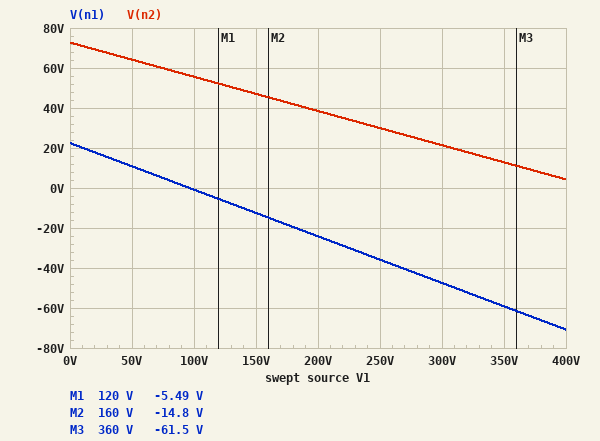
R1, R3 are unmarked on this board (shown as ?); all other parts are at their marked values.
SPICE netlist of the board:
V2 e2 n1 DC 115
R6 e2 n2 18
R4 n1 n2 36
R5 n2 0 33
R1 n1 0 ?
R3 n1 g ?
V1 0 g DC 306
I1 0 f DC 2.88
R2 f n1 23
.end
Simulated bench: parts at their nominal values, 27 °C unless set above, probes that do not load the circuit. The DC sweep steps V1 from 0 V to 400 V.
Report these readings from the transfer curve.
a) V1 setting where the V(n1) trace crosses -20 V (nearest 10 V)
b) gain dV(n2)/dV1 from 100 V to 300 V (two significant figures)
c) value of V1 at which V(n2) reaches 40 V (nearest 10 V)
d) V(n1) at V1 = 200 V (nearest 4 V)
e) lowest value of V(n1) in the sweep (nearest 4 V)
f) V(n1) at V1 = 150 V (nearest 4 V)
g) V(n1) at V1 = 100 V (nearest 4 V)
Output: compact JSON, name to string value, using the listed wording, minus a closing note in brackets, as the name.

{"V1 setting where the V(n1) trace crosses -20 V": "180 V", "gain dV(n2)/dV1 from 100 V to 300 V": "-0.17 V/V", "value of V1 at which V(n2) reaches 40 V": "190 V", "V(n1) at V1 = 200 V": "-24 V", "lowest value of V(n1) in the sweep": "-72 V", "V(n1) at V1 = 150 V": "-12 V", "V(n1) at V1 = 100 V": "0 V"}
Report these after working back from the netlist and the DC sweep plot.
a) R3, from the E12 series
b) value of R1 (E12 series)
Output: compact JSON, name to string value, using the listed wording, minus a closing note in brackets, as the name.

{"R3, from the E12 series": "82 Ω", "value of R1": "56 Ω"}
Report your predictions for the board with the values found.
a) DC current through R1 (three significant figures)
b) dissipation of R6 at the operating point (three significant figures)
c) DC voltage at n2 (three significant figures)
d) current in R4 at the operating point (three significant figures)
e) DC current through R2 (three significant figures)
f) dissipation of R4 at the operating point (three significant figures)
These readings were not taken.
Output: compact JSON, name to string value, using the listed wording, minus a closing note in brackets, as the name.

{"DC current through R1": "873 mA", "dissipation of R6 at the operating point": "116 W", "DC voltage at n2": "20.4 V", "current in R4 at the operating point": "1.92 A", "DC current through R2": "2.88 A", "dissipation of R4 at the operating point": "133 W"}
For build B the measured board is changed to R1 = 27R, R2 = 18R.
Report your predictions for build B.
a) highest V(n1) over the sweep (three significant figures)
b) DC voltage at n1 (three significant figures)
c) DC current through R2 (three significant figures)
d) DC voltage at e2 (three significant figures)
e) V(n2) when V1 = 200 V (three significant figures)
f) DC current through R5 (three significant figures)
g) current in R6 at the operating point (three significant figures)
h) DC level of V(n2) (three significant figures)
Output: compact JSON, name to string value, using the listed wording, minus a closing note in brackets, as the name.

{"highest V(n1) over the sweep": "16.5 V", "DC voltage at n1": "-35.8 V", "DC current through R2": "2.88 A", "DC voltage at e2": "79.2 V", "V(n2) when V1 = 200 V": "43.3 V", "DC current through R5": "909 mA", "current in R6 at the operating point": "2.74 A", "DC level of V(n2)": "30.0 V"}
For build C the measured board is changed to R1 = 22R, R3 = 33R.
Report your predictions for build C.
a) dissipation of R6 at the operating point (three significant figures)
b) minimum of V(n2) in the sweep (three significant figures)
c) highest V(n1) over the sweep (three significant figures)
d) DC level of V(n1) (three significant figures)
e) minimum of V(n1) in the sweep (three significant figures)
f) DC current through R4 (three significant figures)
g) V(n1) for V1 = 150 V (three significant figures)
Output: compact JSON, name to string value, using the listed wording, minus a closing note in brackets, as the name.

{"dissipation of R6 at the operating point": "75.0 W", "minimum of V(n2) in the sweep": "-25.7 V", "highest V(n1) over the sweep": "12.0 V", "DC level of V(n1)": "-82.6 V", "minimum of V(n1) in the sweep": "-112 V", "DC current through R4": "2.17 A", "V(n1) for V1 = 150 V": "-34.4 V"}
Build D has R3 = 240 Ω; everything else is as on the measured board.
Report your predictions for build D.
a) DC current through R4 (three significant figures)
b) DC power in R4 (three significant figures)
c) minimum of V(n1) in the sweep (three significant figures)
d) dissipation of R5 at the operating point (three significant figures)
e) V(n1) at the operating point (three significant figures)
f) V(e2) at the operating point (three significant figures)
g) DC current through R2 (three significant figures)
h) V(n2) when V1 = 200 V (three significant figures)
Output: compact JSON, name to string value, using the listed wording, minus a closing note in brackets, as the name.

{"DC current through R4": "1.58 A", "DC power in R4": "89.7 W", "minimum of V(n1) in the sweep": "-11.1 V", "dissipation of R5 at the operating point": "90.3 W", "V(n1) at the operating point": "-2.23 V", "V(e2) at the operating point": "113 V", "DC current through R2": "2.88 A", "V(n2) when V1 = 200 V": "61.9 V"}
